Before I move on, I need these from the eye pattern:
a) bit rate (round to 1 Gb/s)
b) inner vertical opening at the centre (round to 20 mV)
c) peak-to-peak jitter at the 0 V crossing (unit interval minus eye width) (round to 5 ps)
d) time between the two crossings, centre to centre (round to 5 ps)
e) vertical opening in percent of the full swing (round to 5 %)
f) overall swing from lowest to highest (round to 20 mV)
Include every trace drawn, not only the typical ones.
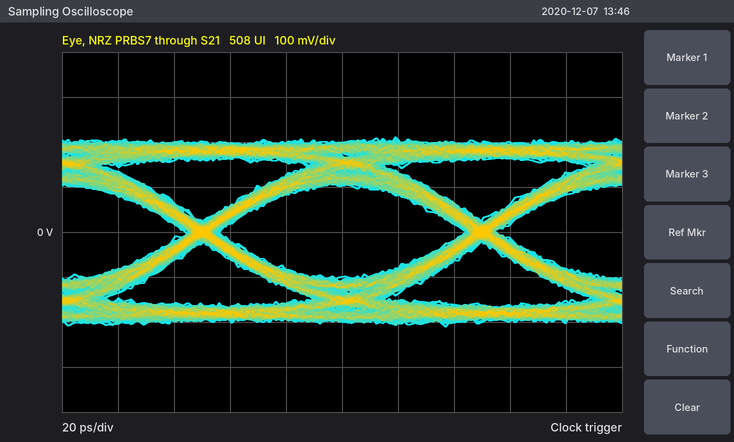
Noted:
10 Gb/s
200 mV
10 ps
100 ps
50 %
420 mV
